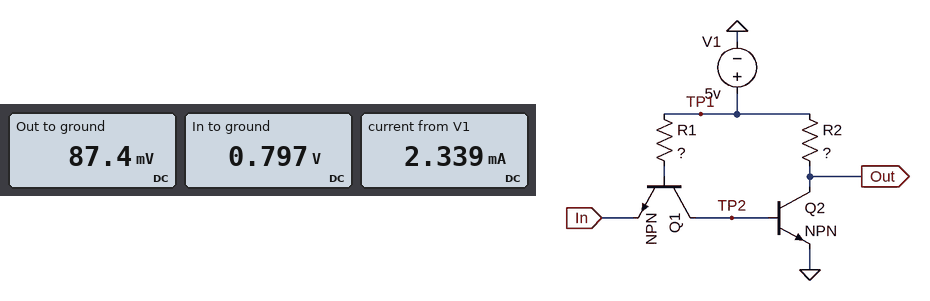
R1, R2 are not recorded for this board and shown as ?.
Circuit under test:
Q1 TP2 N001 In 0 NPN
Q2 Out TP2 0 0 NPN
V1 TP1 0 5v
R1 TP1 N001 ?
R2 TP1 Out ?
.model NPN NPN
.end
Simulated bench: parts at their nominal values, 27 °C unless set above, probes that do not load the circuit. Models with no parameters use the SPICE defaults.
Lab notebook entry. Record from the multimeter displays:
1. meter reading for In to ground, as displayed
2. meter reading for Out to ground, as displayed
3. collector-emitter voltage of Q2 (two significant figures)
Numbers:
0.797 V
87.4 mV
87 mV
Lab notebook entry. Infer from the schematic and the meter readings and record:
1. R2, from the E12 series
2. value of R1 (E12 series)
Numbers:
2.2 kΩ
33 kΩ
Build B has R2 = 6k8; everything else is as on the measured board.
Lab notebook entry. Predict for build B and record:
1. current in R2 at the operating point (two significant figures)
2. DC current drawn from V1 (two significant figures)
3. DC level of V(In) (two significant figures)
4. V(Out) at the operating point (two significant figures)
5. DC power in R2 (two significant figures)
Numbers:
730 µA
830 µA
770 mV
58 mV
3.6 mW
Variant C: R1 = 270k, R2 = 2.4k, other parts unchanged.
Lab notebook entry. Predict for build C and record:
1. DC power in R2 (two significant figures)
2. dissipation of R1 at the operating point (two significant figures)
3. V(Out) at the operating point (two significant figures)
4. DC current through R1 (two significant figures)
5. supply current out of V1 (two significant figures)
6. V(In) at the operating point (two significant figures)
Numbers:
4.2 mW
47 µW
1.8 V
13 µA
1.3 mA
780 mV
